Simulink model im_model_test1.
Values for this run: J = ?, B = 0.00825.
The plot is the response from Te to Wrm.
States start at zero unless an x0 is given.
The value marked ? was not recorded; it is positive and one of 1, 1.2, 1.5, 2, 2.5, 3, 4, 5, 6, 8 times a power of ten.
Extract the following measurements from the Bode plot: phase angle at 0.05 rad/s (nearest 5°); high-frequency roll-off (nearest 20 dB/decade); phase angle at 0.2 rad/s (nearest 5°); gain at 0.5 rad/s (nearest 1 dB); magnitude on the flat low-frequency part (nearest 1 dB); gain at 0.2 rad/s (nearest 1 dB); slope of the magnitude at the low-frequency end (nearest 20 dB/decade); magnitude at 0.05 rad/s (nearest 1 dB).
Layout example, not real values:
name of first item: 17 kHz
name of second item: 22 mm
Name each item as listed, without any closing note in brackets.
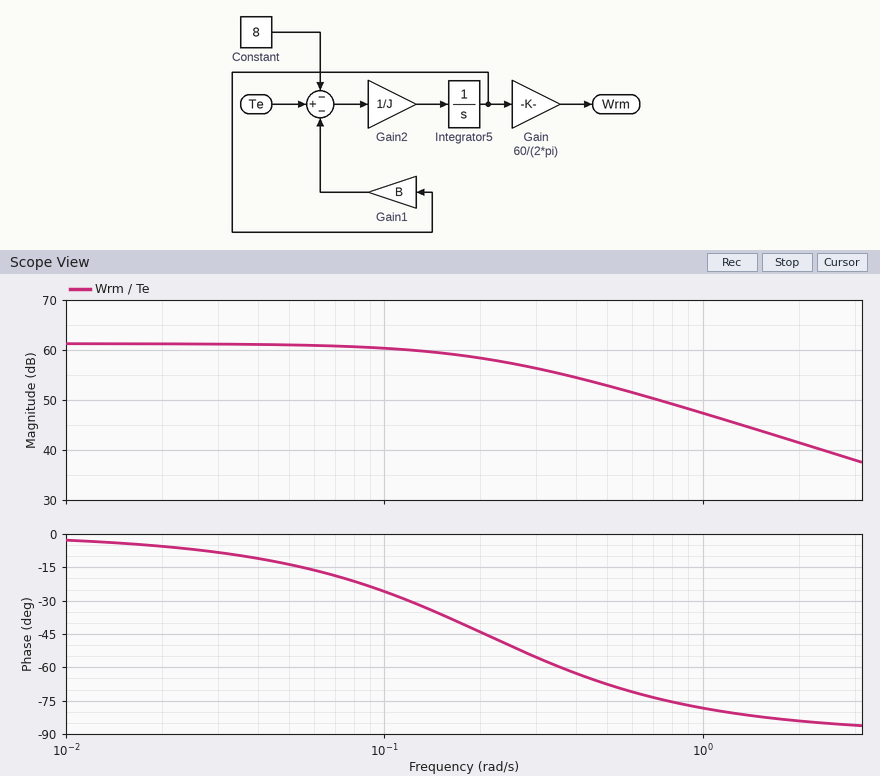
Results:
phase angle at 0.05 rad/s: -15°
high-frequency roll-off: -20 dB/decade
phase angle at 0.2 rad/s: -45°
gain at 0.5 rad/s: 53 dB
magnitude on the flat low-frequency part: 61 dB
gain at 0.2 rad/s: 58 dB
slope of the magnitude at the low-frequency end: 0 dB/decade
magnitude at 0.05 rad/s: 61 dB
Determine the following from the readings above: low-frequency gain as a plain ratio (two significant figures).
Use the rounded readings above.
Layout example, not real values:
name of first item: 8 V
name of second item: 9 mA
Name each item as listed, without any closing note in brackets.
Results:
low-frequency gain as a plain ratio: 1100
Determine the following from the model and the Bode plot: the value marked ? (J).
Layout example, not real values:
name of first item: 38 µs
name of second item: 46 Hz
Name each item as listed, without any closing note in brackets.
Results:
the value marked ?: 0.04
